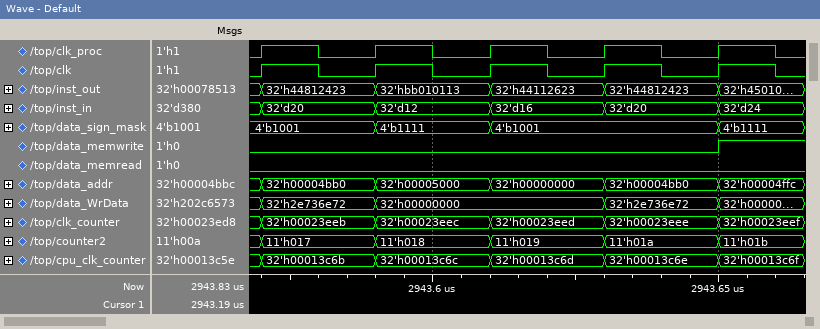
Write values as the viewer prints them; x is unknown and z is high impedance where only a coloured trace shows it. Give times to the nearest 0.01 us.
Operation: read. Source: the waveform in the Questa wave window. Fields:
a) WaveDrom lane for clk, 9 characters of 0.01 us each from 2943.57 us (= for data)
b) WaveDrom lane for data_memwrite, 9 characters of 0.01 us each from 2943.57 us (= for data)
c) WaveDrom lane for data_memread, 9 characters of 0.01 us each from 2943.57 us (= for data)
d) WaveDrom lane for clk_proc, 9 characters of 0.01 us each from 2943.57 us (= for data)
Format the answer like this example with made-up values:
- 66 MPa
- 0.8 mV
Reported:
- {name: 'clk', wave: '101010101'}
- {name: 'data_memwrite', wave: '0.......1'}
- {name: 'data_memread', wave: '0........'}
- {name: 'clk_proc', wave: '101010101'}
